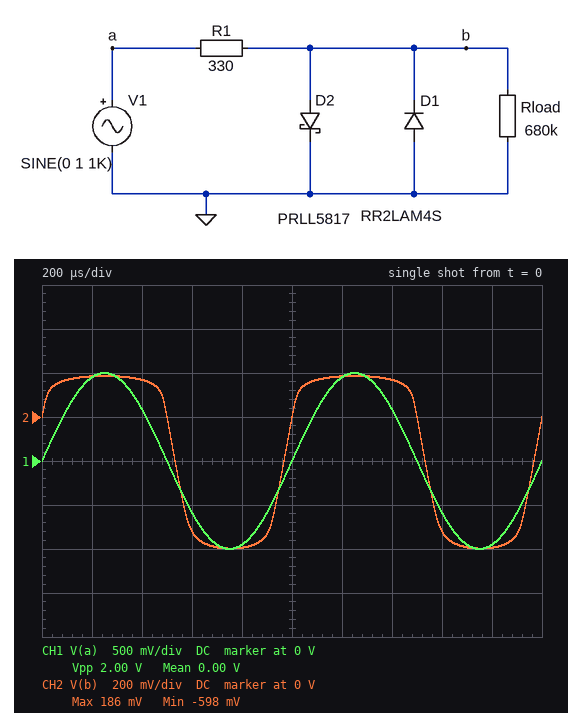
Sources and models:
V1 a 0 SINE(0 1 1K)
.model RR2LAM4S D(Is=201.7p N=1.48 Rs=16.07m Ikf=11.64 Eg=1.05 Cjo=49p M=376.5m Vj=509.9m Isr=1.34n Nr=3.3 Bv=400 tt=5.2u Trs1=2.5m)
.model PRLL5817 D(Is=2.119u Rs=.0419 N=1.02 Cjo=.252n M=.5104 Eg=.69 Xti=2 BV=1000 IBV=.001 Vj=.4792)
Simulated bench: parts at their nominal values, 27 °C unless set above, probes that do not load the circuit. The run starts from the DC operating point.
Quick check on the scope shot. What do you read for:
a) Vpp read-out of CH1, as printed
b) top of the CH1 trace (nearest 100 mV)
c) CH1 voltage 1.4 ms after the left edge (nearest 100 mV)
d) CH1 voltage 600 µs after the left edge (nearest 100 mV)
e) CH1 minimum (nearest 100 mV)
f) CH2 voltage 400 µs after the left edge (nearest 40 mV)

2.00 V
1.0 V
600 mV
-600 mV
-1.0 V
160 mV
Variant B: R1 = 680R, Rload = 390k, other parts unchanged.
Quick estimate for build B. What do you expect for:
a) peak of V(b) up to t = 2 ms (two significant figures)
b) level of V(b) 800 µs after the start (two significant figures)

170 mV
-570 mV
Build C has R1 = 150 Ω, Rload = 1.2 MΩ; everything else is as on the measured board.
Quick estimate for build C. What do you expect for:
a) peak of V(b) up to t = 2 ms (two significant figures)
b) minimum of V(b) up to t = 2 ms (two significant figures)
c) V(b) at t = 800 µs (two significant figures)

210 mV
-630 mV
-620 mV
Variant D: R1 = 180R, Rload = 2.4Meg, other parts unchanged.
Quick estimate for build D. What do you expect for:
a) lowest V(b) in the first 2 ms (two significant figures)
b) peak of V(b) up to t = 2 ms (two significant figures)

-620 mV
200 mV
